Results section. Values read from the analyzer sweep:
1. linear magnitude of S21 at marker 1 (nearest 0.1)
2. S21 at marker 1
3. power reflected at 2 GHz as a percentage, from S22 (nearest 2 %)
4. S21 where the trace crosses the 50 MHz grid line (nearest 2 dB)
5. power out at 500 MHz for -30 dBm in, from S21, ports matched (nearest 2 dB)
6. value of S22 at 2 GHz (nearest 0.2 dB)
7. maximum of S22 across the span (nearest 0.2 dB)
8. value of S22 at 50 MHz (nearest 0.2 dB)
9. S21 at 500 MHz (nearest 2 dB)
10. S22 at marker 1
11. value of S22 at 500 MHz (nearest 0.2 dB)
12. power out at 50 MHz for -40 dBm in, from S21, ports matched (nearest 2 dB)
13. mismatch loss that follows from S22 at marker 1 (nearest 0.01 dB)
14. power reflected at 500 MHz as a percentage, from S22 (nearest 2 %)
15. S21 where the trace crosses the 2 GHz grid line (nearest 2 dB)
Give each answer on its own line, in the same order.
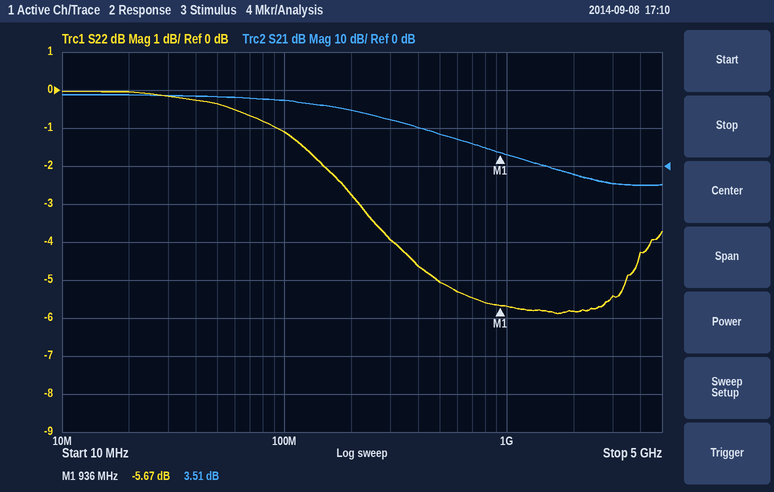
1.5
3.51 dB
26 %
18 dB
-22 dBm
-5.8 dB
0.0 dB
-0.4 dB
8 dB
-5.67 dB
-5.0 dB
-22 dBm
1.37 dB
32 %
-2 dB
